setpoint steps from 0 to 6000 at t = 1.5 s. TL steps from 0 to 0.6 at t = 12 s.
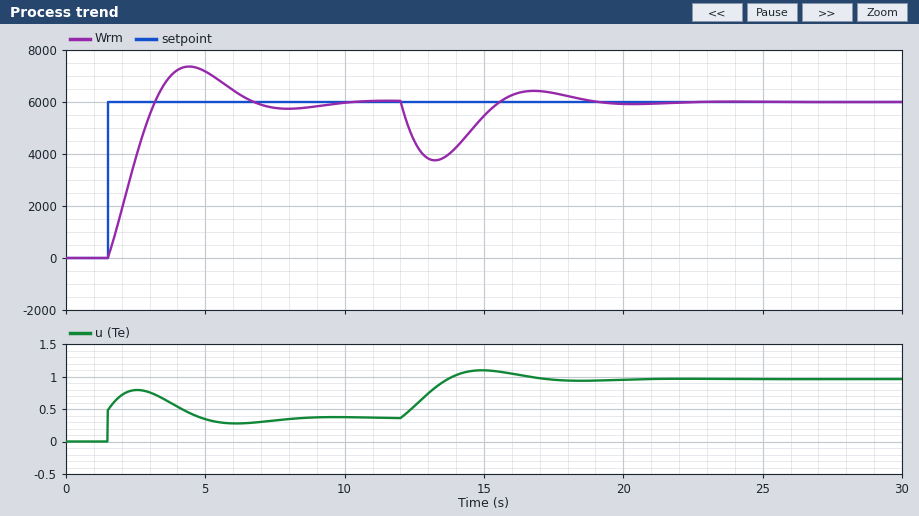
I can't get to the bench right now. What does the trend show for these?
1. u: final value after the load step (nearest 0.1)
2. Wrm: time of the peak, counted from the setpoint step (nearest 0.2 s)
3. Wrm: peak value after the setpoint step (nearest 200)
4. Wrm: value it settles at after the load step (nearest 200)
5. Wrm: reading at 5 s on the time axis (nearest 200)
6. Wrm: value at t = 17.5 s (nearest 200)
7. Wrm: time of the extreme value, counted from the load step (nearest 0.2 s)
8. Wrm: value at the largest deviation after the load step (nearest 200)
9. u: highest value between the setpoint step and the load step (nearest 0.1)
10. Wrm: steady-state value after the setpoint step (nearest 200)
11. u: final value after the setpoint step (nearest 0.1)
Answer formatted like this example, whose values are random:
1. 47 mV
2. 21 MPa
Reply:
1. 1.0
2. 3.0 s
3. 7400
4. 6000
5. 7200
6. 6400
7. 1.2 s
8. 3800
9. 0.8
10. 6000
11. 0.4
